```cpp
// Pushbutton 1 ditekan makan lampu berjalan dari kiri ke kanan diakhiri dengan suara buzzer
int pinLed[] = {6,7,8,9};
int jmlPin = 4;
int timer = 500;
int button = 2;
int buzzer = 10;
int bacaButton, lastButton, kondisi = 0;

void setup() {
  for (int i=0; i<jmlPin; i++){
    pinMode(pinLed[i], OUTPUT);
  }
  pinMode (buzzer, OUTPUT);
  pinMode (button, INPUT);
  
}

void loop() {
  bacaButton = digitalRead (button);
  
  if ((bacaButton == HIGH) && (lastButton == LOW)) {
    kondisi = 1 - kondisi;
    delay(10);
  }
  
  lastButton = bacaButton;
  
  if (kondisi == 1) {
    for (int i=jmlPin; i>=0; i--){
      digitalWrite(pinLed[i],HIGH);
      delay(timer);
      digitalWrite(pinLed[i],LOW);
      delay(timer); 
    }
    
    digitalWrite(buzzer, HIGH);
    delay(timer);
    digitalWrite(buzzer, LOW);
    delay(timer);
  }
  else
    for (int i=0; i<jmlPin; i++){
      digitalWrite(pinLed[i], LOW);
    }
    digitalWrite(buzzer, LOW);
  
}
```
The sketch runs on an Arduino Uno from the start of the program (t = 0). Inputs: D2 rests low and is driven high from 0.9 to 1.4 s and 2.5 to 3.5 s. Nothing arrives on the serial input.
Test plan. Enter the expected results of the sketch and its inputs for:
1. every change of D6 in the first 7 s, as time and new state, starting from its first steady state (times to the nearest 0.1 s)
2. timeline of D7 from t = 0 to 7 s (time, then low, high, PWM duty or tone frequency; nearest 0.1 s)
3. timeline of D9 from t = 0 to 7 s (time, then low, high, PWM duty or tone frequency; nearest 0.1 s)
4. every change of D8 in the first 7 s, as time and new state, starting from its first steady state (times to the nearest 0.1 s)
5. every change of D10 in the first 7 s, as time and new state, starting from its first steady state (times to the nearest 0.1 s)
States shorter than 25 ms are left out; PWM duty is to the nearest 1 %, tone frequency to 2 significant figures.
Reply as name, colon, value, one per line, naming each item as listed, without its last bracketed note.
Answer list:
every change of D6 in the first 7 s, as time and new state, starting from its first steady state: 0 s low; 4.9 s high; 5.4 s low
timeline of D7 from t = 0 to 7 s: 0 s low; 3.9 s high; 4.4 s low
timeline of D9 from t = 0 to 7 s: 0 s low; 1.9 s high; 2.4 s low
every change of D8 in the first 7 s, as time and new state, starting from its first steady state: 0 s low; 2.9 s high; 3.4 s low
every change of D10 in the first 7 s, as time and new state, starting from its first steady state: 0 s low; 5.9 s high; 6.4 s low
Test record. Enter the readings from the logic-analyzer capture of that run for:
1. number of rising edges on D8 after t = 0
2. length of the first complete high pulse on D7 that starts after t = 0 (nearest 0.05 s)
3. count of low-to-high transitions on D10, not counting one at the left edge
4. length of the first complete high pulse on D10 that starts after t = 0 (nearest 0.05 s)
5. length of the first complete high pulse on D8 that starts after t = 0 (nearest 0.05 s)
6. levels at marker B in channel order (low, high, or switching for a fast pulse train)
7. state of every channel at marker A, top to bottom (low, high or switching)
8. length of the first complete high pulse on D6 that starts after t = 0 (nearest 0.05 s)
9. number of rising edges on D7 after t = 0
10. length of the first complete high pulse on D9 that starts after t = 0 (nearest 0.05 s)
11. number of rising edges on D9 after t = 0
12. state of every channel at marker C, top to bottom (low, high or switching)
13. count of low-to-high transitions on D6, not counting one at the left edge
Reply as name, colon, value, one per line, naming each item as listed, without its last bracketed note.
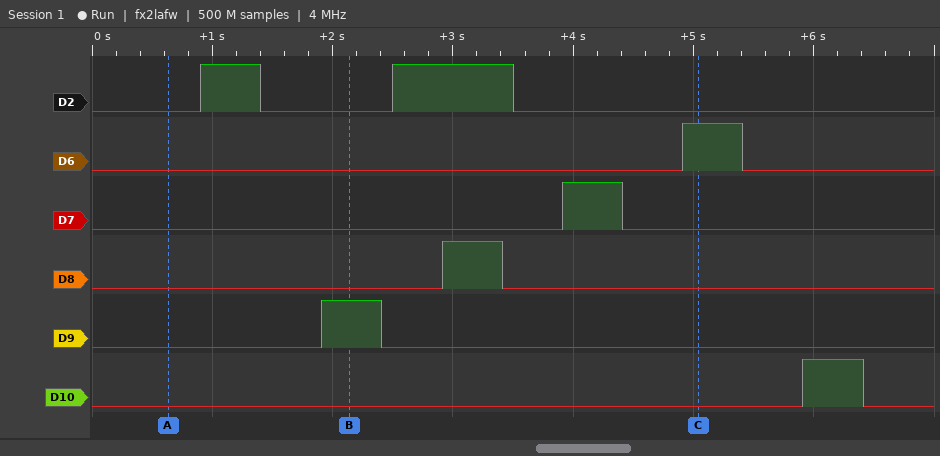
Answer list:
number of rising edges on D8 after t = 0: 1
length of the first complete high pulse on D7 that starts after t = 0: 0.50 s
count of low-to-high transitions on D10, not counting one at the left edge: 1
length of the first complete high pulse on D10 that starts after t = 0: 0.50 s
length of the first complete high pulse on D8 that starts after t = 0: 0.50 s
levels at marker B in channel order: D2 low, D6 low, D7 low, D8 low, D9 high, D10 low
state of every channel at marker A, top to bottom: D2 low, D6 low, D7 low, D8 low, D9 low, D10 low
length of the first complete high pulse on D6 that starts after t = 0: 0.50 s
number of rising edges on D7 after t = 0: 1
length of the first complete high pulse on D9 that starts after t = 0: 0.50 s
number of rising edges on D9 after t = 0: 1
state of every channel at marker C, top to bottom: D2 low, D6 high, D7 low, D8 low, D9 low, D10 low
count of low-to-high transitions on D6, not counting one at the left edge: 1
